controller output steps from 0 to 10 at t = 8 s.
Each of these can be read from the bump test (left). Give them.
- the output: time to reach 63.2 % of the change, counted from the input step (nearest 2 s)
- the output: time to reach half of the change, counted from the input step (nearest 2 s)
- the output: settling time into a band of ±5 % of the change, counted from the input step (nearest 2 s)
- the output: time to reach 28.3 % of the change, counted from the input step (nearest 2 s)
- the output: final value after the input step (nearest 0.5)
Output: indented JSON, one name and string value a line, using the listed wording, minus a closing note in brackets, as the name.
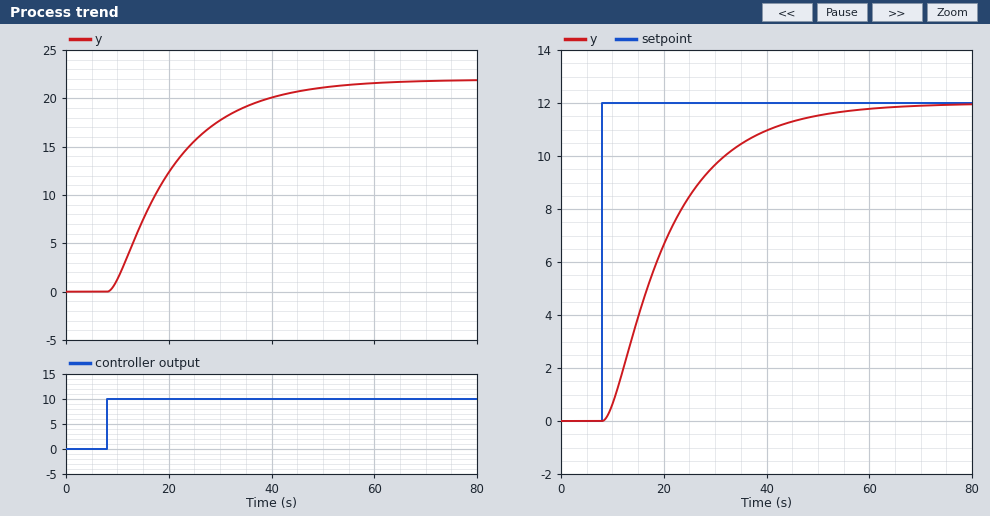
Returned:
{
  "the output: time to reach 63.2 % of the change, counted from the input step": "14 s",
  "the output: time to reach half of the change, counted from the input step": "10 s",
  "the output: settling time into a band of ±5 % of the change, counted from the input step": "38 s",
  "the output: time to reach 28.3 % of the change, counted from the input step": "6 s",
  "the output: final value after the input step": "22.0"
}
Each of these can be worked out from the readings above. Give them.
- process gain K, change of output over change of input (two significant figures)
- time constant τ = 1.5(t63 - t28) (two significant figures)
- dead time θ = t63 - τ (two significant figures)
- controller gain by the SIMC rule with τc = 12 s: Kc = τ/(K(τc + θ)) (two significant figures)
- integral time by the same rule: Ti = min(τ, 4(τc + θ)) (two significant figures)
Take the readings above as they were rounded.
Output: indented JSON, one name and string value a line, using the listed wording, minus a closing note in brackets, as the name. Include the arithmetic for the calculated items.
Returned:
{
  "process gain K, change of output over change of input": "(22 - 0) / 10 = 2.2",
  "time constant τ = 1.5(t63 - t28)": "1.5 × (14 - 6) = 12 s",
  "dead time θ = t63 - τ": "14 - 12 = 2.0 s",
  "controller gain by the SIMC rule with τc = 12 s: Kc = τ/(K(τc + θ))": "12 / (2.2 × (12 + 2)) = 0.39",
  "integral time by the same rule: Ti = min(τ, 4(τc + θ))": "min(12, 4 × (12 + 2)) = 12 s"
}
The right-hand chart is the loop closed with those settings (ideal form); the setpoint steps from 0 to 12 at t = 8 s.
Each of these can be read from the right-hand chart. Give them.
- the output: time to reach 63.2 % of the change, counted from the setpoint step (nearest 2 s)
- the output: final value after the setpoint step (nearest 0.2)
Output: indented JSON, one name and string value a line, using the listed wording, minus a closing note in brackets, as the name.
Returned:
{
  "the output: time to reach 63.2 % of the change, counted from the setpoint step": "14 s",
  "the output: final value after the setpoint step": "12.0"
}
